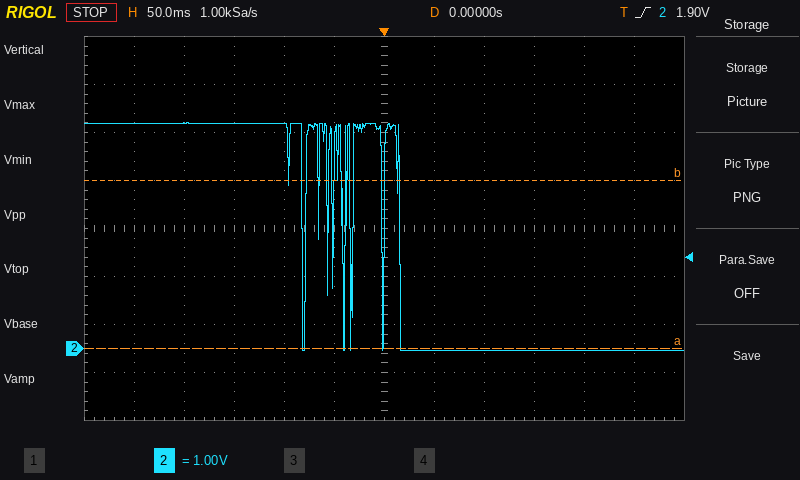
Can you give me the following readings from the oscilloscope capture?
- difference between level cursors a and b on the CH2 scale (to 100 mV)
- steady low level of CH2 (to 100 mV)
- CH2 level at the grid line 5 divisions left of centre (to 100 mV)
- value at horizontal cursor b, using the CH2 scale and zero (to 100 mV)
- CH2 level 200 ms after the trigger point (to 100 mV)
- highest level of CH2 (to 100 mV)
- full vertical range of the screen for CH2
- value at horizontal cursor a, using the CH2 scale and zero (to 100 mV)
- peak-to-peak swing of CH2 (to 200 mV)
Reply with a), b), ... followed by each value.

a) 3.5 V
b) 0.0 V
c) 4.7 V
d) 3.5 V
e) 0.0 V
f) 4.7 V
g) 8 V
h) 0.0 V
i) 4.8 V
